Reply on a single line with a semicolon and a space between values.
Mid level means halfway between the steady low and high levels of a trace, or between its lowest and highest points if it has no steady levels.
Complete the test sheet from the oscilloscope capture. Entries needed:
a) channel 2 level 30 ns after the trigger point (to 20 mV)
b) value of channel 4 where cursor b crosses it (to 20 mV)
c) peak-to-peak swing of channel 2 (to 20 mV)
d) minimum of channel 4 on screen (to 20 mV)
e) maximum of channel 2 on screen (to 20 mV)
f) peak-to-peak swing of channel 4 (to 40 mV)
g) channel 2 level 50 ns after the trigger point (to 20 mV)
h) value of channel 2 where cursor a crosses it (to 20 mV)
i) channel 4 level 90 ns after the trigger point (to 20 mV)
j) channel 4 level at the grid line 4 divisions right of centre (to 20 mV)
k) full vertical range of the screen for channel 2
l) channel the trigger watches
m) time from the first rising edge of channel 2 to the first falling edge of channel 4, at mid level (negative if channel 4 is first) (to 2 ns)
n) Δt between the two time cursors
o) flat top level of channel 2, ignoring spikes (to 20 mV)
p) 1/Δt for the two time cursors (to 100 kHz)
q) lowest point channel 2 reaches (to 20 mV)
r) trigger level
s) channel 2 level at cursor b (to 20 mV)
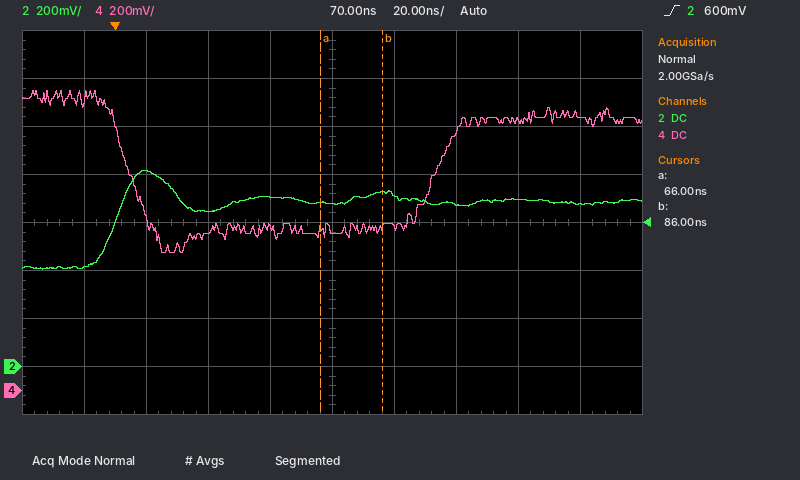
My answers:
640 mV; 680 mV; 420 mV; 580 mV; 820 mV; 680 mV; 700 mV; 680 mV; 680 mV; 1.14 V; 1.6 V; channel 2; +6 ns; 20 ns; 680 mV; 50.0 MHz; 400 mV; 600 mV; 720 mV
